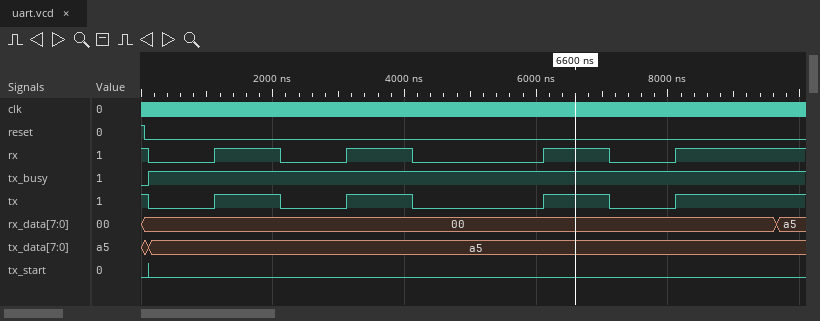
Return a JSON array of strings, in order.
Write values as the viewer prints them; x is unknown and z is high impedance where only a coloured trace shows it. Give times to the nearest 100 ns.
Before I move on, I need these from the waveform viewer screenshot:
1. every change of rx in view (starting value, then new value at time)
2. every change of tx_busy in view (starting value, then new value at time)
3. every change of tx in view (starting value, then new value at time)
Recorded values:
["1, 0 at 100 ns, 1 at 1100 ns, 0 at 2100 ns, 1 at 3100 ns, 0 at 4100 ns, 1 at 6100 ns, 0 at 7100 ns, 1 at 8100 ns", "0, 1 at 100 ns", "1, 0 at 100 ns, 1 at 1100 ns, 0 at 2100 ns, 1 at 3100 ns, 0 at 4100 ns, 1 at 6100 ns, 0 at 7100 ns, 1 at 8100 ns"]
